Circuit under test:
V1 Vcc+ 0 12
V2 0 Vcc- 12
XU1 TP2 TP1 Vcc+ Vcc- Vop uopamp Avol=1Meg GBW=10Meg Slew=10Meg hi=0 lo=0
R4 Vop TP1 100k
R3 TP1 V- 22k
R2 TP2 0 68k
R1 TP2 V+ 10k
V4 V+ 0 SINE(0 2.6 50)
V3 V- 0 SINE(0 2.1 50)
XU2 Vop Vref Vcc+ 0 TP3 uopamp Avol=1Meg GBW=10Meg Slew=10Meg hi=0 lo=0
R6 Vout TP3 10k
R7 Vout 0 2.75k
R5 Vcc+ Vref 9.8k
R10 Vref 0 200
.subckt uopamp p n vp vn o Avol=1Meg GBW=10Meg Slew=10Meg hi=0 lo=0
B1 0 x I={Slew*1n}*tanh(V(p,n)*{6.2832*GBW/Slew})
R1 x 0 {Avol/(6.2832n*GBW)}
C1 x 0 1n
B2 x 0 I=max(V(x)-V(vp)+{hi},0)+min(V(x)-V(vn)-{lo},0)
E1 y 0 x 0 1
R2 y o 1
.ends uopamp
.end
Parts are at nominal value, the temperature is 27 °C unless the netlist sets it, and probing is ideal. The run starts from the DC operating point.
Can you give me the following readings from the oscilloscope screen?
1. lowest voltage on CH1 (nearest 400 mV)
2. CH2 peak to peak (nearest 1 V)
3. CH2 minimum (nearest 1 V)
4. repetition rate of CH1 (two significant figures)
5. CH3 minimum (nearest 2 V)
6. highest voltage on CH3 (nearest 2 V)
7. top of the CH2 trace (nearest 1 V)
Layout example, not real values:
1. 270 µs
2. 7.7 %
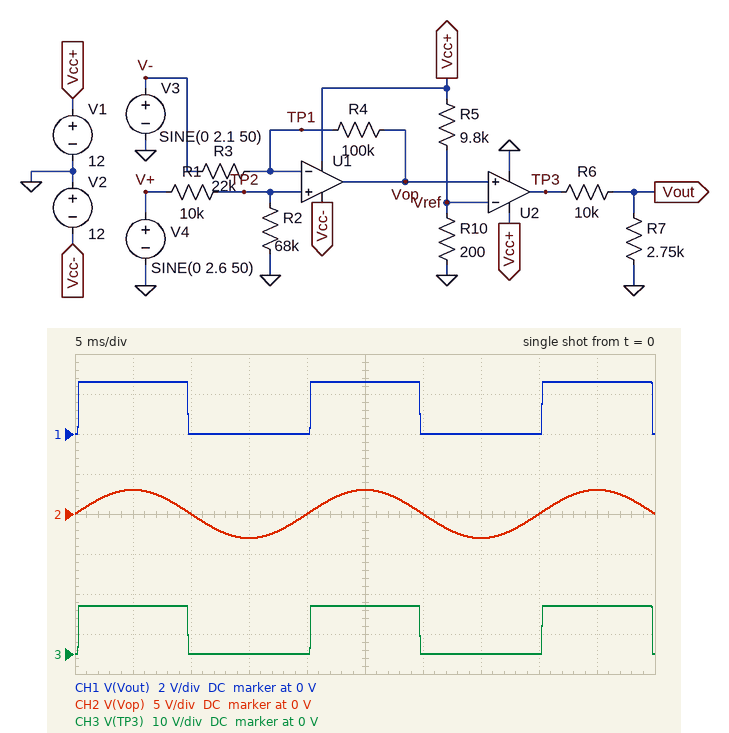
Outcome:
1. 0 V
2. 6 V
3. -3 V
4. 50 Hz
5. 0 V
6. 12 V
7. 3 V
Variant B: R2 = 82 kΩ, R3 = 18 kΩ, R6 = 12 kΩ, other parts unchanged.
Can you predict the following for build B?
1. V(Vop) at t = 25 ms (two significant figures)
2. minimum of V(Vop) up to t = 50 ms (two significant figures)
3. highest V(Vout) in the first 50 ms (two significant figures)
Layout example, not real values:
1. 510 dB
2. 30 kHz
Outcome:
1. 3.5 V
2. -3.5 V
3. 2.2 V
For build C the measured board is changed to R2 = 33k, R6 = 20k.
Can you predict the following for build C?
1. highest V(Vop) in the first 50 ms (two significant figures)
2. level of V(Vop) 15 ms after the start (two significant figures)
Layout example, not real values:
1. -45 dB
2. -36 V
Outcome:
1. 1.5 V
2. -1.5 V
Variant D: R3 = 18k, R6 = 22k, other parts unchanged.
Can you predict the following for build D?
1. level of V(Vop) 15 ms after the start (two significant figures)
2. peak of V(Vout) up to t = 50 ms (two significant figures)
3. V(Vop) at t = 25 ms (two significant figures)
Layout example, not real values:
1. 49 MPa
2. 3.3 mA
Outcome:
1. -3.2 V
2. 1.3 V
3. 3.2 V
